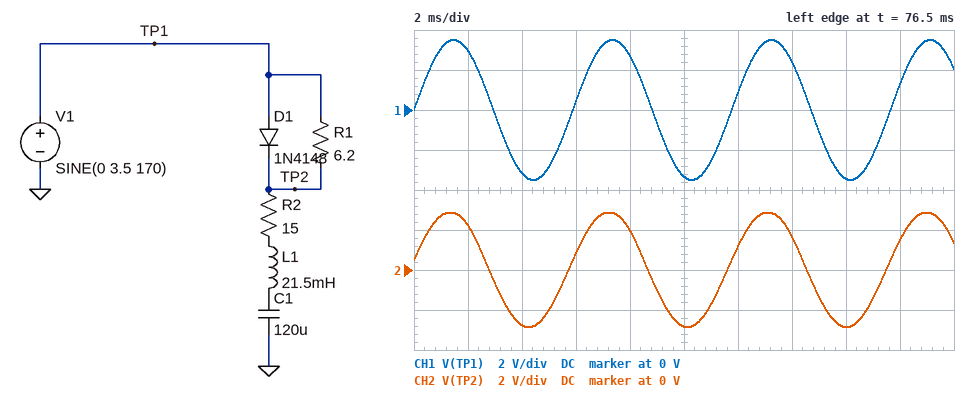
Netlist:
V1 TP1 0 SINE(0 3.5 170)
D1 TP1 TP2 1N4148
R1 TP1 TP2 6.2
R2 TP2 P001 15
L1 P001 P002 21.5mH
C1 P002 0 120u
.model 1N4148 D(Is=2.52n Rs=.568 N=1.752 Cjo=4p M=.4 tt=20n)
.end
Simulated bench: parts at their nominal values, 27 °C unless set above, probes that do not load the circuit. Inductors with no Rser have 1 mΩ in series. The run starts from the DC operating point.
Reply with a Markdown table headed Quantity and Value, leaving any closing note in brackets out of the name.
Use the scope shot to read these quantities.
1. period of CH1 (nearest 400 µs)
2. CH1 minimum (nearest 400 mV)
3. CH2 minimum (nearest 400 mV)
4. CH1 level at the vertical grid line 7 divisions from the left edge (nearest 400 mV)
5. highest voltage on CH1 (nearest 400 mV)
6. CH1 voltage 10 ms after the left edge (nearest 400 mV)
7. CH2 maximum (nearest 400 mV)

| Quantity | Value |
|---|---|
| period of CH1 | 6.0 ms |
| CH1 minimum | -3.6 V |
| CH2 minimum | -2.8 V |
| CH1 level at the vertical grid line 7 divisions from the left edge | 2.4 V |
| highest voltage on CH1 | 3.6 V |
| CH1 voltage 10 ms after the left edge | -3.2 V |
| CH2 maximum | 2.8 V |
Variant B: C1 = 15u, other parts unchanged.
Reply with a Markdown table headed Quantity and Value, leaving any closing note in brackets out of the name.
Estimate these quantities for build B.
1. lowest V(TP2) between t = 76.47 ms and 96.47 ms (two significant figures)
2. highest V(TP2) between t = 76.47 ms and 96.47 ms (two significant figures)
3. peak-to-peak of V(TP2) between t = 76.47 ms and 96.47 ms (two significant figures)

| Quantity | Value |
|---|---|
| lowest V(TP2) between t = 76.47 ms and 96.47 ms | -3.3 V |
| highest V(TP2) between t = 76.47 ms and 96.47 ms | 3.3 V |
| peak-to-peak of V(TP2) between t = 76.47 ms and 96.47 ms | 6.6 V |
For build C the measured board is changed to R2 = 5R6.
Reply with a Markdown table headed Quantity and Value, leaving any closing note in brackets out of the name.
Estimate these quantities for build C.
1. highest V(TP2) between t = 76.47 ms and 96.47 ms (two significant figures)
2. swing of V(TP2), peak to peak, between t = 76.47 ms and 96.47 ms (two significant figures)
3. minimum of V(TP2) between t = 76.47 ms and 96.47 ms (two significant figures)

| Quantity | Value |
|---|---|
| highest V(TP2) between t = 76.47 ms and 96.47 ms | 3.0 V |
| swing of V(TP2), peak to peak, between t = 76.47 ms and 96.47 ms | 5.9 V |
| minimum of V(TP2) between t = 76.47 ms and 96.47 ms | -3.0 V |
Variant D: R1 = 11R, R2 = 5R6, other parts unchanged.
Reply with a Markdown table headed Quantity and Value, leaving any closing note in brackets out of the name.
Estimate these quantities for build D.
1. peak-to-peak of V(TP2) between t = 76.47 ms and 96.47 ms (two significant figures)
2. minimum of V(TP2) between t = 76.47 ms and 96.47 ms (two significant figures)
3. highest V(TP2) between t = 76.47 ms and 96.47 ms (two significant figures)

| Quantity | Value |
|---|---|
| peak-to-peak of V(TP2) between t = 76.47 ms and 96.47 ms | 5.3 V |
| minimum of V(TP2) between t = 76.47 ms and 96.47 ms | -2.6 V |
| highest V(TP2) between t = 76.47 ms and 96.47 ms | 2.7 V |
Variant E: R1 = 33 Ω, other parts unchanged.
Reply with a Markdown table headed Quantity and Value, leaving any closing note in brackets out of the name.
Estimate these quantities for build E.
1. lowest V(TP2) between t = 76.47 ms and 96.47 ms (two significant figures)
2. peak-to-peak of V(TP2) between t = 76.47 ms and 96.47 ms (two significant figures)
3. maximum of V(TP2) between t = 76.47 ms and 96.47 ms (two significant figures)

| Quantity | Value |
|---|---|
| lowest V(TP2) between t = 76.47 ms and 96.47 ms | -1.2 V |
| peak-to-peak of V(TP2) between t = 76.47 ms and 96.47 ms | 3.9 V |
| maximum of V(TP2) between t = 76.47 ms and 96.47 ms | 2.7 V |
